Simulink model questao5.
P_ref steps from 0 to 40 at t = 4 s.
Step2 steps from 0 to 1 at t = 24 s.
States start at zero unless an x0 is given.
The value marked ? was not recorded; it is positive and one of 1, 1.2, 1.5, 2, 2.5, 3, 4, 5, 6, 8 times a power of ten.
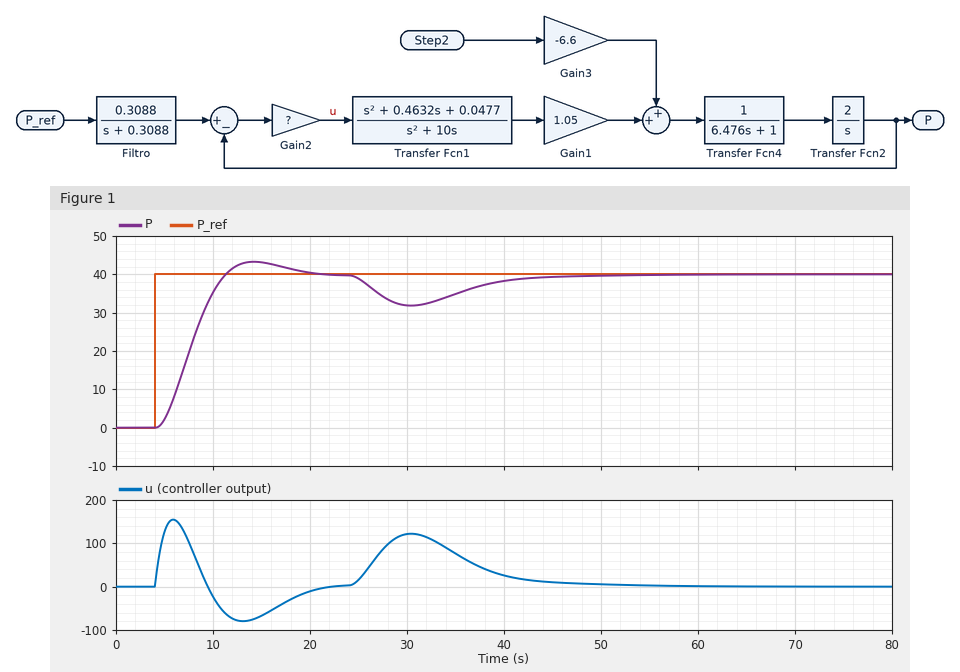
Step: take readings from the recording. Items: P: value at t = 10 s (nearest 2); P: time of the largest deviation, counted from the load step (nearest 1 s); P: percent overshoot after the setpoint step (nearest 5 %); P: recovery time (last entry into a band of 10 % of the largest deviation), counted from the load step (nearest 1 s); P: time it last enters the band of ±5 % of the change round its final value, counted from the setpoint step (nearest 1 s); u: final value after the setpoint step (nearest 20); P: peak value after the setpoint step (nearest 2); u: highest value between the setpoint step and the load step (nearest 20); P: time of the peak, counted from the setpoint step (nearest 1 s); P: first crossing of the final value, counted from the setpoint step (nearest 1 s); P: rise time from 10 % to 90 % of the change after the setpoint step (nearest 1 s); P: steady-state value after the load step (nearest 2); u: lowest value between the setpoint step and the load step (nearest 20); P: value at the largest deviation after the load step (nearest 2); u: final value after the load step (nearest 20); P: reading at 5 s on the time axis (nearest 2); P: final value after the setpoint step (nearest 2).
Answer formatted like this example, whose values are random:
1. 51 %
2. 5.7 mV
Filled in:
1. 36
2. 6 s
3. 10 %
4. 20 s
5. 13 s
6. 0
7. 44
8. 160
9. 10 s
10. 7 s
11. 5 s
12. 40
13. -80
14. 32
15. 0
16. 2
17. 40
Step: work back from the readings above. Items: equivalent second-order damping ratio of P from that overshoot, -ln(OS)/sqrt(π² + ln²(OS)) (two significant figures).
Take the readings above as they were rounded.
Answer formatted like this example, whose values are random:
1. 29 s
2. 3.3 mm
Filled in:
1. 0.59
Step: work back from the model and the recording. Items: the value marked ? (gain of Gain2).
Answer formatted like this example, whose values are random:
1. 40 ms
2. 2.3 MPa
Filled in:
1. 15
